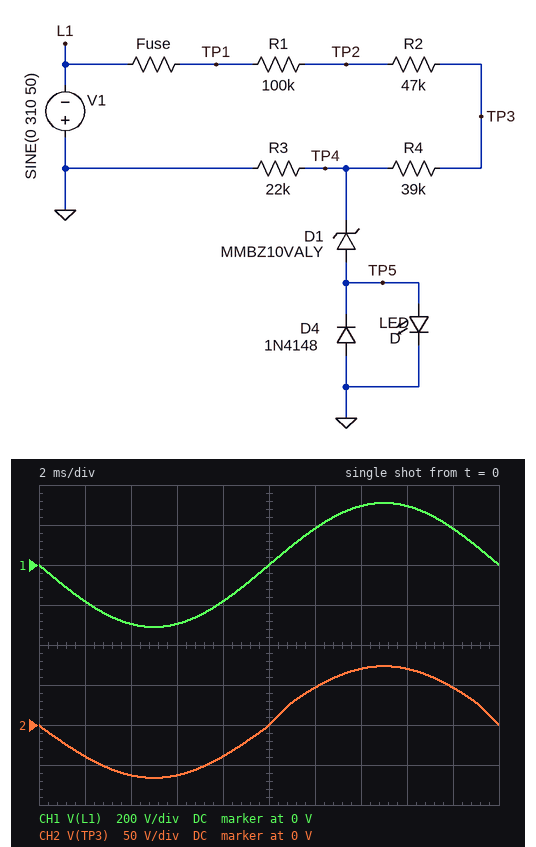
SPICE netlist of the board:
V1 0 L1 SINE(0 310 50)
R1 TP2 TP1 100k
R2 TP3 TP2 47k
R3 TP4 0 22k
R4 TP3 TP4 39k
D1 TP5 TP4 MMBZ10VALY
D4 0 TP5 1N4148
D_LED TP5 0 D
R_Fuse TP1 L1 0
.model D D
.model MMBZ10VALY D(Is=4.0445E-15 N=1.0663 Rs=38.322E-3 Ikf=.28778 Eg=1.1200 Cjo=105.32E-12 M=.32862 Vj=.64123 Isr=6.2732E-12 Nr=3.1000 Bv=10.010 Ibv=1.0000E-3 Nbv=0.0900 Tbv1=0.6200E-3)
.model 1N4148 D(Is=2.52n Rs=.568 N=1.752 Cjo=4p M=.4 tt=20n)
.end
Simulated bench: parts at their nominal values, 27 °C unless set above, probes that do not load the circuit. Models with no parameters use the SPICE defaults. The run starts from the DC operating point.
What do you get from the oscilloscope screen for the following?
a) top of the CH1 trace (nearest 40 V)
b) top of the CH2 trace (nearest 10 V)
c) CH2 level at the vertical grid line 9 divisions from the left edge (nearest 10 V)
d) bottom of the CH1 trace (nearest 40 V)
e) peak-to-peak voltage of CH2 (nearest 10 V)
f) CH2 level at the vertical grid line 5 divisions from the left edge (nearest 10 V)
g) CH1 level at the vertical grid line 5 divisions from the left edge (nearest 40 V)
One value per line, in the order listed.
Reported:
320 V
70 V
50 V
-320 V
140 V
0 V
0 V
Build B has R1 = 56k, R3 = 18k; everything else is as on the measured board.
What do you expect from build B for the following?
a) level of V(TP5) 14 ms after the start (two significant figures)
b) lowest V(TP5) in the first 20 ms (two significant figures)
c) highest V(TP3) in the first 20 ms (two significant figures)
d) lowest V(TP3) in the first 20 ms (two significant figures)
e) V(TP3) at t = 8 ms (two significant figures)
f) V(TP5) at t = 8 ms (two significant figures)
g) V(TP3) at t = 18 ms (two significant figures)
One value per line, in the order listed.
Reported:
660 mV
-620 mV
93 V
-86 V
-51 V
-590 mV
58 V
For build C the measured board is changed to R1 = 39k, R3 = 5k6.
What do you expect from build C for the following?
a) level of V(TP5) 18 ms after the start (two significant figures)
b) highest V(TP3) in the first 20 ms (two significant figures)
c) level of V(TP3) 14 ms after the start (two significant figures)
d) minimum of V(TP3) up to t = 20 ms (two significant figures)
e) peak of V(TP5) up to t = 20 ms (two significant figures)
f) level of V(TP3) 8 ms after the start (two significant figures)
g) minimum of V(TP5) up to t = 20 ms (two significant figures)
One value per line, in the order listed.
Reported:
-190 mV
100 V
99 V
-98 V
640 mV
-58 V
-620 mV
